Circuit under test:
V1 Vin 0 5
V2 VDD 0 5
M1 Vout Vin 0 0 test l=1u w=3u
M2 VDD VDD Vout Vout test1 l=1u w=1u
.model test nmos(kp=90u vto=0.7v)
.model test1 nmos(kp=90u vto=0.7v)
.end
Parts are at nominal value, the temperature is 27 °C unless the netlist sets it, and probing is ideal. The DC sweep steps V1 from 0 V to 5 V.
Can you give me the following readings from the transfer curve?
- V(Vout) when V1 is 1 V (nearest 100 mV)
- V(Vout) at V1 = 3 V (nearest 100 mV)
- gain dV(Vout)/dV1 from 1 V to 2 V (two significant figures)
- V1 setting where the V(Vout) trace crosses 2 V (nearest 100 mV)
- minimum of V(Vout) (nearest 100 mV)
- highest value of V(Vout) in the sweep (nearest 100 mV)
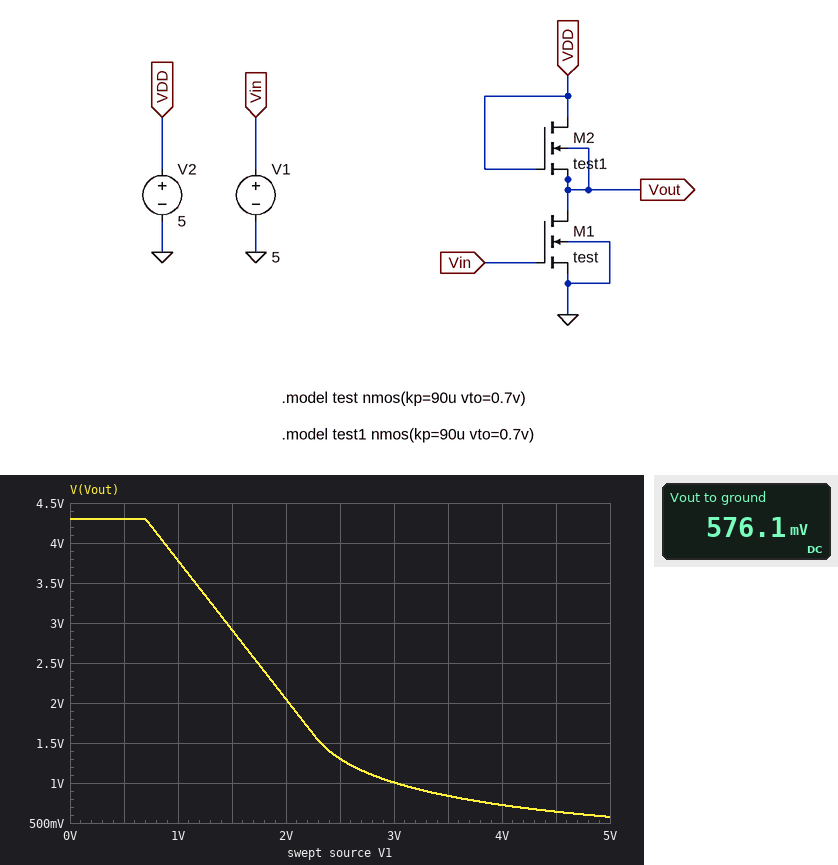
3.8 V
1.0 V
-1.7 V/V
2.0 V
600 mV
4.3 V
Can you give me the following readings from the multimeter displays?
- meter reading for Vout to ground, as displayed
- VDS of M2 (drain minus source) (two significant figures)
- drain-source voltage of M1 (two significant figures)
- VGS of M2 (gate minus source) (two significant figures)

576.1 mV
4.4 V
580 mV
4.4 V
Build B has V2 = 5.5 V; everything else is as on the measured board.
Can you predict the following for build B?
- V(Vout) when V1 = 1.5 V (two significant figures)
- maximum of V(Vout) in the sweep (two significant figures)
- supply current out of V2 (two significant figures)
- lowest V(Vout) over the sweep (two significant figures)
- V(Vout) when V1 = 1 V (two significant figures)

3.4 V
4.8 V
750 µA
710 mV
4.3 V
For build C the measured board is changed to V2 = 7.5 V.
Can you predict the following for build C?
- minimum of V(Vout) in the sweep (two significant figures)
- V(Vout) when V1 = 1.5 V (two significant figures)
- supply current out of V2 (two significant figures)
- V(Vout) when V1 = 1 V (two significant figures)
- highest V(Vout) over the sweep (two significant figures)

1.4 V
5.4 V
1.3 mA
6.3 V
6.8 V
